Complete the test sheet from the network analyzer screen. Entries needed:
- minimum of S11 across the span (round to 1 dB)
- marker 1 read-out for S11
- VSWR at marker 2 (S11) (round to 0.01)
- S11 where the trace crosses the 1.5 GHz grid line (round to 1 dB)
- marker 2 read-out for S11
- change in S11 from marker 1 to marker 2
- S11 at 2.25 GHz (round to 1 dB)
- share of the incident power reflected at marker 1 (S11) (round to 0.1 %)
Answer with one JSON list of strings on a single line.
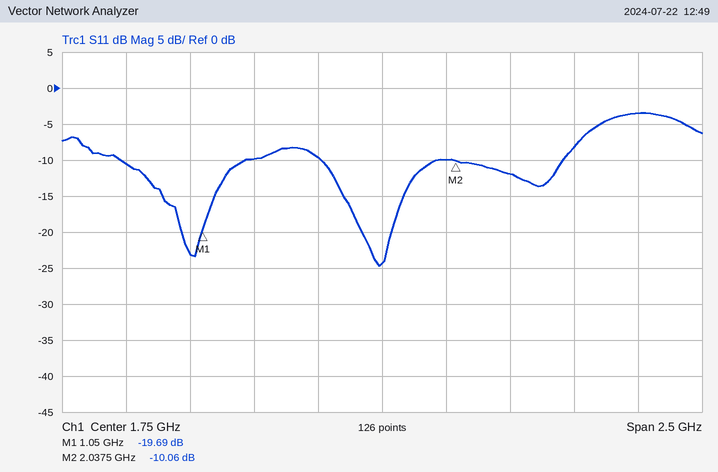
["-25 dB", "-19.69 dB", "1.92", "-10 dB", "-10.06 dB", "9.63 dB", "-12 dB", "1.1 %"]
